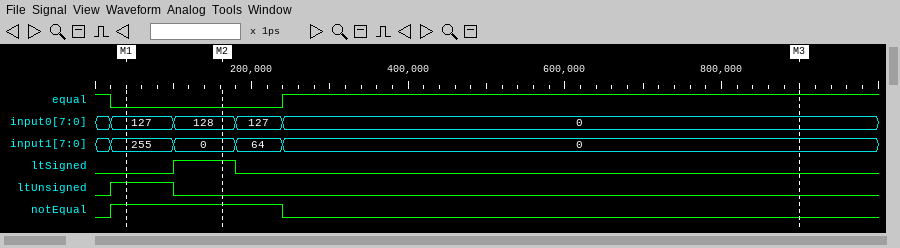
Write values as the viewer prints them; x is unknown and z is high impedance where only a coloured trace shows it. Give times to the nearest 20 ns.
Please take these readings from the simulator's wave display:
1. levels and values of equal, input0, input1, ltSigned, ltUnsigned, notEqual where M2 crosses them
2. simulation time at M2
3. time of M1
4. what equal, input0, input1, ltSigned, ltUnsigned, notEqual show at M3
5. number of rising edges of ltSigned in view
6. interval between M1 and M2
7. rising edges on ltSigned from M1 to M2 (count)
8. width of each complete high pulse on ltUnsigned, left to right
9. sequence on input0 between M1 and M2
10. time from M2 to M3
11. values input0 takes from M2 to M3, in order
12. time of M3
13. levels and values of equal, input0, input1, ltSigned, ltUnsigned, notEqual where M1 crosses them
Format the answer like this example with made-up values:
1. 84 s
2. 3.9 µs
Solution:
1. equal=0, input0=128, input1=0, ltSigned=1, ltUnsigned=0, notEqual=1
2. 160 ns
3. 40 ns
4. equal=1, input0=0, input1=0, ltSigned=0, ltUnsigned=0, notEqual=0
5. 1
6. 120 ns
7. 1
8. 80 ns
9. 127, 128
10. 740 ns
11. 128, 127, 0
12. 900 ns
13. equal=0, input0=127, input1=255, ltSigned=0, ltUnsigned=1, notEqual=1
